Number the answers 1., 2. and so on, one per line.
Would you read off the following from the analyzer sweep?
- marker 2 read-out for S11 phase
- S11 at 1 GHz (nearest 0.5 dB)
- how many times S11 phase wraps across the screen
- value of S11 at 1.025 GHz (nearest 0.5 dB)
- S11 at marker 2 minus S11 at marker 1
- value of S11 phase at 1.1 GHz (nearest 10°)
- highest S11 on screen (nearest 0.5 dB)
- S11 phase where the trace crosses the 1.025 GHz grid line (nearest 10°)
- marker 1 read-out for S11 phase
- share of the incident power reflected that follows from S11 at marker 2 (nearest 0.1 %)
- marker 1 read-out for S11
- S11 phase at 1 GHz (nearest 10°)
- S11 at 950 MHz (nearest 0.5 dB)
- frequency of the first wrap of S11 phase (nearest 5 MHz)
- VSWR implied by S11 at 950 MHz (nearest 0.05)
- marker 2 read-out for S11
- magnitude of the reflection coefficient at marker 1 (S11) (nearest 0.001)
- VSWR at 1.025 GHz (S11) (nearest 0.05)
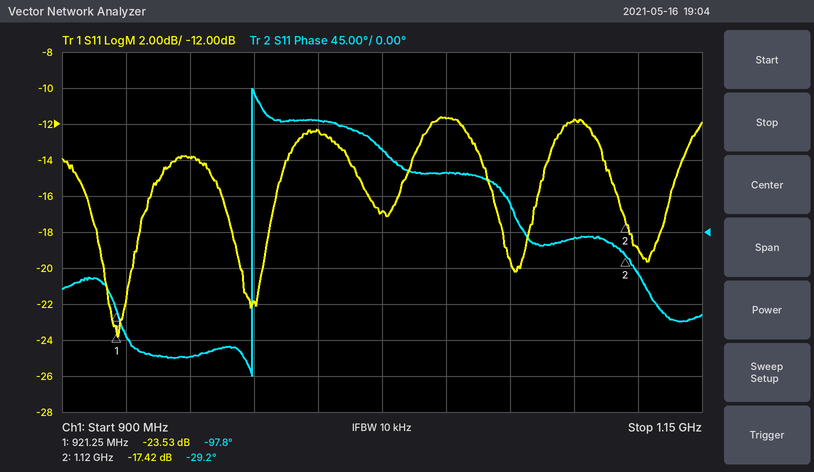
1. -29.2°
2. -12.5 dB
3. 1
4. -17.0 dB
5. 6.11 dB
6. -10°
7. -11.5 dB
8. 100°
9. -97.8°
10. 1.8 %
11. -23.53 dB
12. 140°
13. -14.0 dB
14. 975 MHz
15. 1.50
16. -17.42 dB
17. 0.067
18. 1.35
